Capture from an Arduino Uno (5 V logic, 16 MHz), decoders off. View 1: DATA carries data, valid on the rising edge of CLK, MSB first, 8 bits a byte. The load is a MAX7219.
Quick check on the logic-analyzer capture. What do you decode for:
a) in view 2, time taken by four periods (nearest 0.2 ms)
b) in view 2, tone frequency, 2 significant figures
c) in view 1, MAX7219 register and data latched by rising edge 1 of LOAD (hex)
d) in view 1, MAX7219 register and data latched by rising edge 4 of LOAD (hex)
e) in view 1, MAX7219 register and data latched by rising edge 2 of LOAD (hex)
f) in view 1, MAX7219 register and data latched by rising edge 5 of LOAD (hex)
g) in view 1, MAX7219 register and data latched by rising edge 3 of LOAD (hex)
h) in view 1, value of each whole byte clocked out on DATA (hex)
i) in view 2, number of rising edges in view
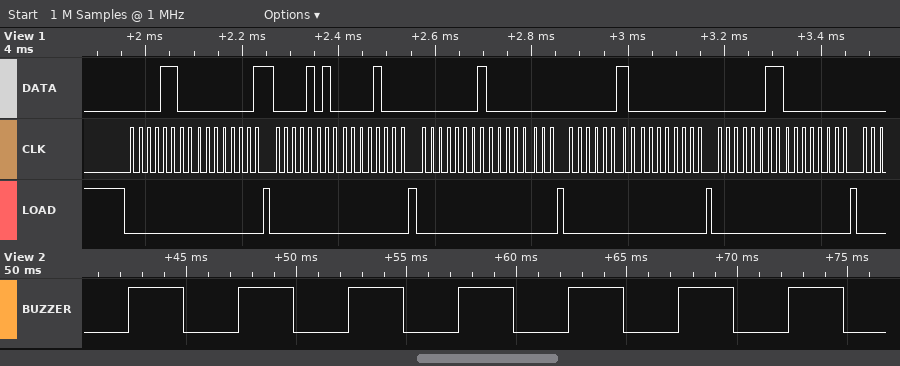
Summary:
20.0 ms
200 Hz
register 0xC, data 0x01
register 0x2, data 0x00
register 0xA, data 0x08
register 0x3, data 0x00
register 0x1, data 0x00
0x0C 0x01 0x0A 0x08 0x01 0x00 0x02 0x00 0x03 0x00
7
